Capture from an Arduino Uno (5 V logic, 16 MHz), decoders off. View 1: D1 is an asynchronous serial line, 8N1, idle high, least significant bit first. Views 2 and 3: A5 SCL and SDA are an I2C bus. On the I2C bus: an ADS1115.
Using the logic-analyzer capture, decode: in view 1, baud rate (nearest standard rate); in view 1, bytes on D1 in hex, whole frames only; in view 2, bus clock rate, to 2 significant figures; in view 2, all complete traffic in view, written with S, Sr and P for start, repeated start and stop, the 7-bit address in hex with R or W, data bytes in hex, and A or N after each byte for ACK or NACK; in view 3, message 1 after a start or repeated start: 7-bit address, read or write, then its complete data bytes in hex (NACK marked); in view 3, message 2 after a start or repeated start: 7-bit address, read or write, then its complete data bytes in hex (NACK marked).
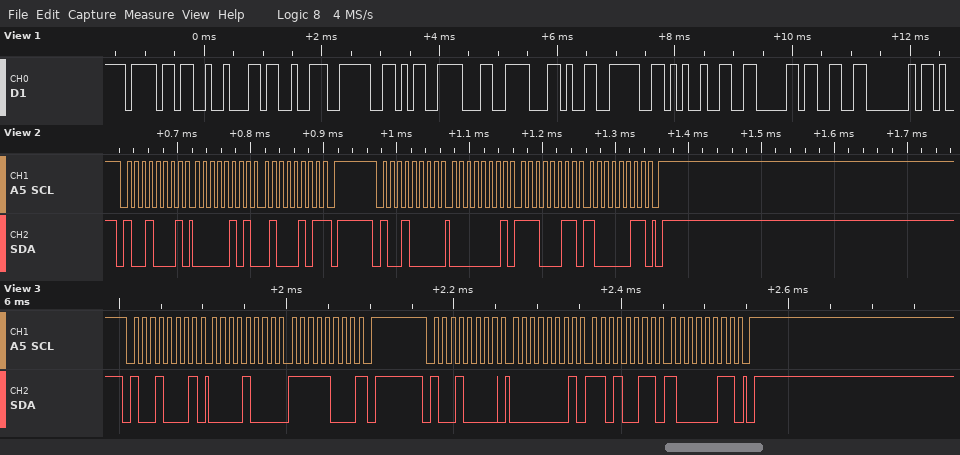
9600 baud
6F 12 93 3E CD CC 2C 3E 25 06 33 40
100 kHz
S 48R A 05 A 45 N P S 48W A 01 A E3 A 83 A P
0x48 read: 08 F8 NACK
0x48 write: 01 D3 83
